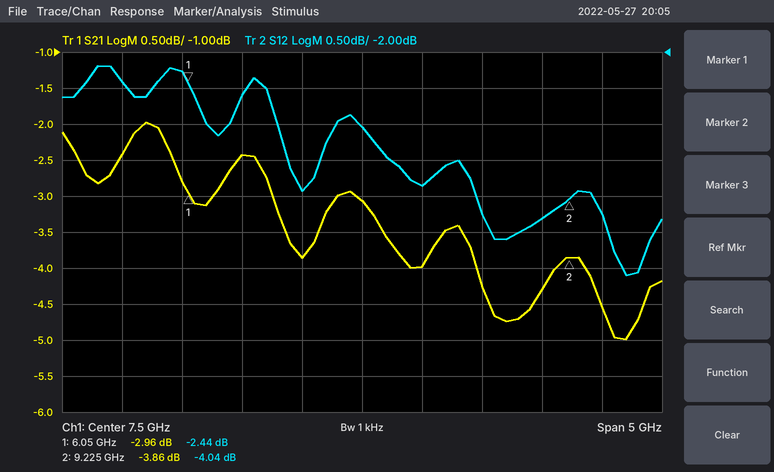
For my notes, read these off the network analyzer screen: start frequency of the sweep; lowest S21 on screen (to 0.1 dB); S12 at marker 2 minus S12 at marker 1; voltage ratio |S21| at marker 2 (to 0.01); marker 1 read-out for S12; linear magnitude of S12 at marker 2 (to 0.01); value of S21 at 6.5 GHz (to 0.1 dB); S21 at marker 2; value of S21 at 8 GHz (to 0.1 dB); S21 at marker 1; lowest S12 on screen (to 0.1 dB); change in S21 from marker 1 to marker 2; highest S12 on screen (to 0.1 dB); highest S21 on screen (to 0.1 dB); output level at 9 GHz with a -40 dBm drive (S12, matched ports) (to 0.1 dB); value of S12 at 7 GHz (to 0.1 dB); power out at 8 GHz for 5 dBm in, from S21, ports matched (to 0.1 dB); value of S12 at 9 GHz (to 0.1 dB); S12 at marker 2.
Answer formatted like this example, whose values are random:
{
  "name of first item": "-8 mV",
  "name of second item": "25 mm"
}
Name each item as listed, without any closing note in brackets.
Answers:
{
  "start frequency of the sweep": "5 GHz",
  "lowest S21 on screen": "-5.0 dB",
  "S12 at marker 2 minus S12 at marker 1": "-1.60 dB",
  "voltage ratio |S21| at marker 2": "0.64",
  "marker 1 read-out for S12": "-2.44 dB",
  "linear magnitude of S12 at marker 2": "0.63",
  "value of S21 at 6.5 GHz": "-2.4 dB",
  "S21 at marker 2": "-3.86 dB",
  "value of S21 at 8 GHz": "-4.0 dB",
  "S21 at marker 1": "-2.96 dB",
  "lowest S12 on screen": "-5.1 dB",
  "change in S21 from marker 1 to marker 2": "-0.90 dB",
  "highest S12 on screen": "-2.2 dB",
  "highest S21 on screen": "-2.0 dB",
  "output level at 9 GHz with a -40 dBm drive (S12, matched ports)": "-44.3 dBm",
  "value of S12 at 7 GHz": "-3.9 dB",
  "power out at 8 GHz for 5 dBm in, from S21, ports matched": "1.0 dBm",
  "value of S12 at 9 GHz": "-4.3 dB",
  "S12 at marker 2": "-4.04 dB"
}
